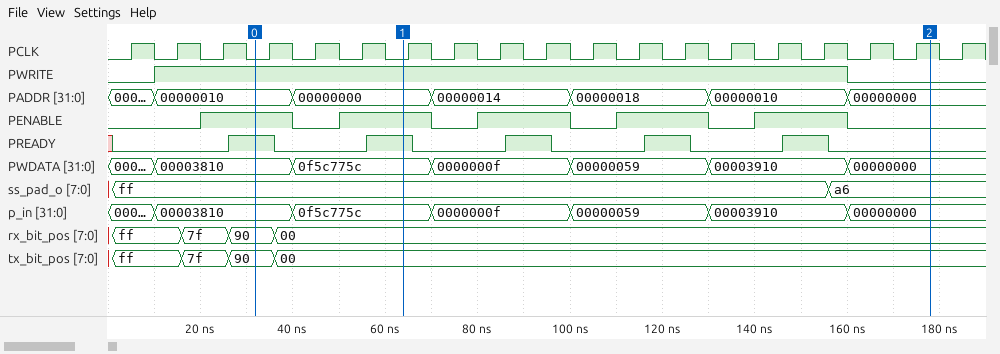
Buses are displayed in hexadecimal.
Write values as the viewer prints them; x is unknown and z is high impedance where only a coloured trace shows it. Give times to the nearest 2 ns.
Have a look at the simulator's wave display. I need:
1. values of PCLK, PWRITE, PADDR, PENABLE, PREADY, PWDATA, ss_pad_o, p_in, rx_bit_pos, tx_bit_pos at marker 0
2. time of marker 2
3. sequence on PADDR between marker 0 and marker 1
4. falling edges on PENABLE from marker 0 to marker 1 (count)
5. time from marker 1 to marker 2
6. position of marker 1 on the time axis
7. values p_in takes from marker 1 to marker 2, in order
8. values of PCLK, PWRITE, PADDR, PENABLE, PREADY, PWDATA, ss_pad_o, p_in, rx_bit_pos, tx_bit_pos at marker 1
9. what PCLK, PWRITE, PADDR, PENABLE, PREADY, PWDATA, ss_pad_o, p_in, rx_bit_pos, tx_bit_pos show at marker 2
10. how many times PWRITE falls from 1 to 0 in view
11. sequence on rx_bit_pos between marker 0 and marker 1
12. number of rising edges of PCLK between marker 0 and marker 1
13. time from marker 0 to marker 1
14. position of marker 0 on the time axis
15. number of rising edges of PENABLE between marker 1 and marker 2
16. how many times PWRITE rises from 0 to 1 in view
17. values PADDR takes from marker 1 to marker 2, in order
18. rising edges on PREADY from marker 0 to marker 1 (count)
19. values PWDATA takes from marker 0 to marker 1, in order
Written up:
PCLK=0, PWRITE=1, PADDR=00000010, PENABLE=1, PREADY=1, PWDATA=00003810, ss_pad_o=ff, p_in=00003810, rx_bit_pos=90, tx_bit_pos=90
178 ns
00000010, 00000000
1
114 ns
64 ns
0f5c775c, 0000000f, 00000059, 00003910, 00000000
PCLK=0, PWRITE=1, PADDR=00000000, PENABLE=1, PREADY=1, PWDATA=0f5c775c, ss_pad_o=ff, p_in=0f5c775c, rx_bit_pos=00, tx_bit_pos=00
PCLK=1, PWRITE=0, PADDR=00000000, PENABLE=0, PREADY=0, PWDATA=00000000, ss_pad_o=a6, p_in=00000000, rx_bit_pos=00, tx_bit_pos=00
1
90, 00
3
32 ns
32 ns
3
1
00000000, 00000014, 00000018, 00000010, 00000000
1
00003810, 0f5c775c
